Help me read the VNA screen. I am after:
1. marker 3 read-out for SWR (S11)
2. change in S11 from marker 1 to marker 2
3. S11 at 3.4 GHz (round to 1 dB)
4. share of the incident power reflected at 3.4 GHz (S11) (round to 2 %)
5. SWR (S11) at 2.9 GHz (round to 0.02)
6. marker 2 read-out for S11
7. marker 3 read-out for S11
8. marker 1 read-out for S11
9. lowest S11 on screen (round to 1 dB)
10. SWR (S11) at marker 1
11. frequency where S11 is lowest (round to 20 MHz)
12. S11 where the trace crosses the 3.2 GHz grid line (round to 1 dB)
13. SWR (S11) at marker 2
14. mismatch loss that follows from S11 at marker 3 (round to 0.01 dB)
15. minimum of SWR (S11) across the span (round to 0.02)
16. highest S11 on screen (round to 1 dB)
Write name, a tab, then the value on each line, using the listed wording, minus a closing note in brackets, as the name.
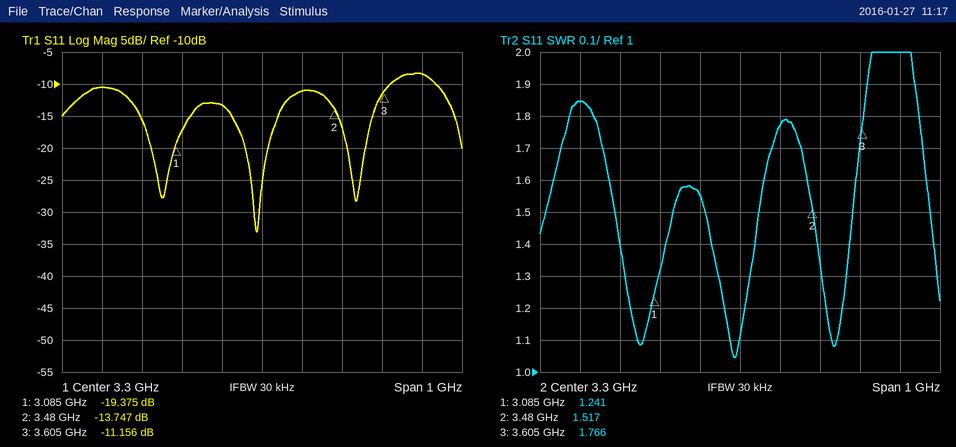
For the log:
marker 3 read-out for SWR	1.766
change in S11 from marker 1 to marker 2	5.628 dB
S11 at 3.4 GHz	-11 dB
share of the incident power reflected at 3.4 GHz (S11)	8 %
SWR (S11) at 2.9 GHz	1.84
marker 2 read-out for S11	-13.747 dB
marker 3 read-out for S11	-11.156 dB
marker 1 read-out for S11	-19.375 dB
lowest S11 on screen	-33 dB
SWR (S11) at marker 1	1.241
frequency where S11 is lowest	3.28 GHz
S11 where the trace crosses the 3.2 GHz grid line	-13 dB
SWR (S11) at marker 2	1.517
mismatch loss that follows from S11 at marker 3	0.35 dB
minimum of SWR (S11) across the span	1.04
highest S11 on screen	-8 dB
